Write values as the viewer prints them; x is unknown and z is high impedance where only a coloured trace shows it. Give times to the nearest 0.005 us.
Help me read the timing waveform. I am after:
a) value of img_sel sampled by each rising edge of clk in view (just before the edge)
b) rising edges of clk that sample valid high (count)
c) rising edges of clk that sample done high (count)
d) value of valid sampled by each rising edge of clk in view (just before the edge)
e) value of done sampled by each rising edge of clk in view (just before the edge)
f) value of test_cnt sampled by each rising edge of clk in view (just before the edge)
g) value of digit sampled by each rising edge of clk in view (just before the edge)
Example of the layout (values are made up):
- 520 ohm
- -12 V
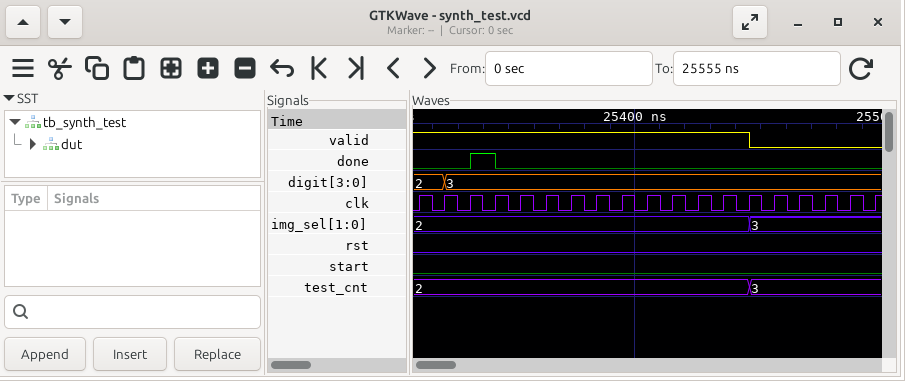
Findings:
- 2, 2, 2, 2, 2, 2, 2, 2, 2, 2, 2, 2, 2, 2, 3, 3, 3, 3, 3
- 14
- 1
- 1 1 1 1 1 1 1 1 1 1 1 1 1 1 0 0 0 0 0
- 0 0 0 1 0 0 0 0 0 0 0 0 0 0 0 0 0 0 0
- 2, 2, 2, 2, 2, 2, 2, 2, 2, 2, 2, 2, 2, 2, 3, 3, 3, 3, 3
- 2, 2, 3, 3, 3, 3, 3, 3, 3, 3, 3, 3, 3, 3, 3, 3, 3, 3, 3
